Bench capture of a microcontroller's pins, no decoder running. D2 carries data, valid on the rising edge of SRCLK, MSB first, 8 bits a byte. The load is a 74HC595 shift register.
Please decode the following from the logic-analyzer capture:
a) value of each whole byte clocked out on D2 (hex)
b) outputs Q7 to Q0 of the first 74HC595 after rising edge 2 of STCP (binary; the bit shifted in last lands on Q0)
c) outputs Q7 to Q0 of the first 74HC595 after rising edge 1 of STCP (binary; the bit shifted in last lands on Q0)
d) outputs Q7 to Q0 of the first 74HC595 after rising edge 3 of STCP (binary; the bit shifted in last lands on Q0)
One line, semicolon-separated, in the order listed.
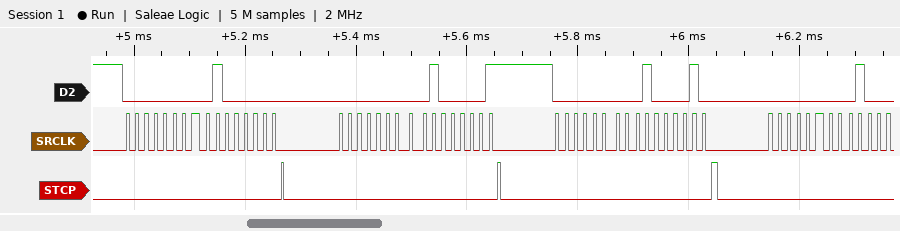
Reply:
0x00 0x40 0x00 0x41 0x00 0x42 0x00; 01000001; 01000000; 01000010
